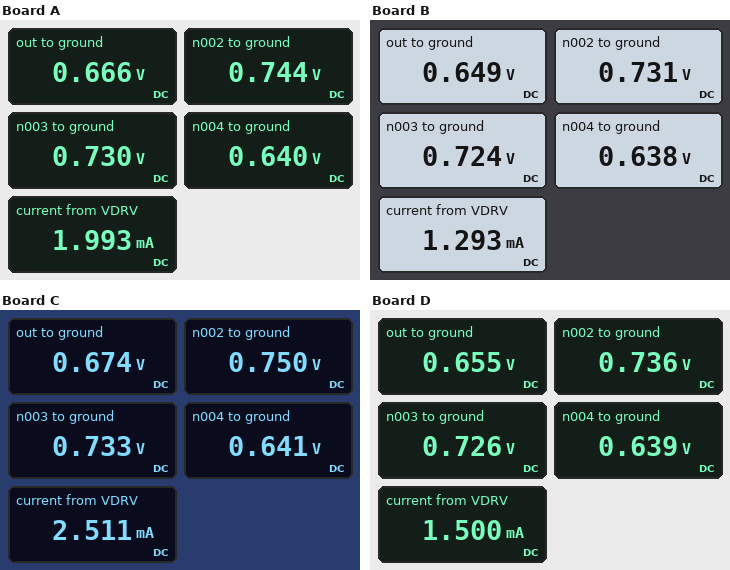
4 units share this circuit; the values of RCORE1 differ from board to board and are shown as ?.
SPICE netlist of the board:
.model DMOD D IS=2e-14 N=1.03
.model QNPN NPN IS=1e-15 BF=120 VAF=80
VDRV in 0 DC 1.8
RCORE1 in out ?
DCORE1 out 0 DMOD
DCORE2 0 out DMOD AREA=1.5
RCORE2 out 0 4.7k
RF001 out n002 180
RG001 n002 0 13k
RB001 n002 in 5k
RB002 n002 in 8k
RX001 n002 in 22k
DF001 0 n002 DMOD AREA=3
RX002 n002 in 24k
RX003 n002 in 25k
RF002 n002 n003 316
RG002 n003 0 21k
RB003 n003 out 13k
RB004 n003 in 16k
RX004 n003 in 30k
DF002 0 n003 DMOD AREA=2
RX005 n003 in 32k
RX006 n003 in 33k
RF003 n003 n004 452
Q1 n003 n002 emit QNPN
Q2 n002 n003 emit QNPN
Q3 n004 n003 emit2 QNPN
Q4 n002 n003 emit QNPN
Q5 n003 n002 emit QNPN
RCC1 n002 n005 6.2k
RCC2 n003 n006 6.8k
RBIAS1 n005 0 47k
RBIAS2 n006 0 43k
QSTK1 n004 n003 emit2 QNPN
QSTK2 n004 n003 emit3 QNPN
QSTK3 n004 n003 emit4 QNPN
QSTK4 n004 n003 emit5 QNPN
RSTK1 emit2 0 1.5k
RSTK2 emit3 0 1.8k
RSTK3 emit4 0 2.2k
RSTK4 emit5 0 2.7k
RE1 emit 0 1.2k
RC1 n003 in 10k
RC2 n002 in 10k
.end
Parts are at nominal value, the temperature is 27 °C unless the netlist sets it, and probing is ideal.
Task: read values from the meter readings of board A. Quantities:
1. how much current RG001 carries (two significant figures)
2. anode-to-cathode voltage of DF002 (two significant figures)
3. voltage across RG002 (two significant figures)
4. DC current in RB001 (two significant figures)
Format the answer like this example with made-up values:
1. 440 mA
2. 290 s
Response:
1. 57 µA
2. -730 mV
3. 730 mV
4. 210 µA
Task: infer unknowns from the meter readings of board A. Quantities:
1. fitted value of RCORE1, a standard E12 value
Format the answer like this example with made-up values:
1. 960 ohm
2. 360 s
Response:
1. 1 kΩ
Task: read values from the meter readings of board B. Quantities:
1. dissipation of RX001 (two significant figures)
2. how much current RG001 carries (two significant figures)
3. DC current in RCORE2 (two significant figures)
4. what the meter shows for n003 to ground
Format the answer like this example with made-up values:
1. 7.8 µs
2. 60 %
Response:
1. 52 µW
2. 56 µA
3. 140 µA
4. 0.724 V
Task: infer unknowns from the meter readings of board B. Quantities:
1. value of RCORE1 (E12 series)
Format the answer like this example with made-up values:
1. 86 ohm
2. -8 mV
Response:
1. 2.7 kΩ
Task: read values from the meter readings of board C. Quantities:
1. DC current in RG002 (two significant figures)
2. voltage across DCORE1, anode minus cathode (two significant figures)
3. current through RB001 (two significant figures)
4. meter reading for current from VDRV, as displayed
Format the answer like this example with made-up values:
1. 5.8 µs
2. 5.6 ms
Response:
1. 35 µA
2. 670 mV
3. 210 µA
4. 2.511 mA
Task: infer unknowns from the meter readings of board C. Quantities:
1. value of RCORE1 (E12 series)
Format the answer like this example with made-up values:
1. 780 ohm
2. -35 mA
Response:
1. 680 Ω
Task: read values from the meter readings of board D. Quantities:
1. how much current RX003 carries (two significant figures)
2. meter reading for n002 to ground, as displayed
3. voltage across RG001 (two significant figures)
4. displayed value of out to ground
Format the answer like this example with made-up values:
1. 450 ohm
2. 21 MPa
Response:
1. 43 µA
2. 0.736 V
3. 740 mV
4. 0.655 V
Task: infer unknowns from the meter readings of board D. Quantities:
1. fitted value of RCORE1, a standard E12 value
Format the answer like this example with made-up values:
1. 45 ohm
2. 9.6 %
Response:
1. 1.8 kΩ
